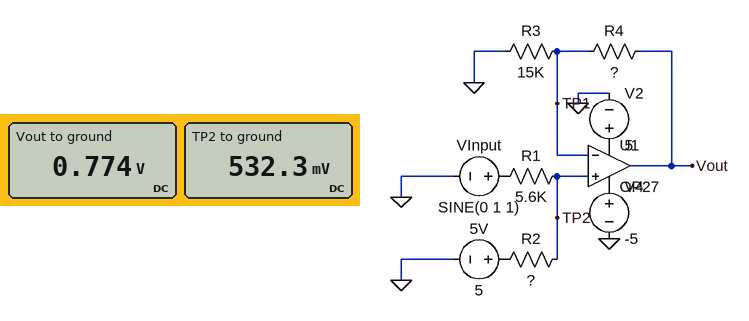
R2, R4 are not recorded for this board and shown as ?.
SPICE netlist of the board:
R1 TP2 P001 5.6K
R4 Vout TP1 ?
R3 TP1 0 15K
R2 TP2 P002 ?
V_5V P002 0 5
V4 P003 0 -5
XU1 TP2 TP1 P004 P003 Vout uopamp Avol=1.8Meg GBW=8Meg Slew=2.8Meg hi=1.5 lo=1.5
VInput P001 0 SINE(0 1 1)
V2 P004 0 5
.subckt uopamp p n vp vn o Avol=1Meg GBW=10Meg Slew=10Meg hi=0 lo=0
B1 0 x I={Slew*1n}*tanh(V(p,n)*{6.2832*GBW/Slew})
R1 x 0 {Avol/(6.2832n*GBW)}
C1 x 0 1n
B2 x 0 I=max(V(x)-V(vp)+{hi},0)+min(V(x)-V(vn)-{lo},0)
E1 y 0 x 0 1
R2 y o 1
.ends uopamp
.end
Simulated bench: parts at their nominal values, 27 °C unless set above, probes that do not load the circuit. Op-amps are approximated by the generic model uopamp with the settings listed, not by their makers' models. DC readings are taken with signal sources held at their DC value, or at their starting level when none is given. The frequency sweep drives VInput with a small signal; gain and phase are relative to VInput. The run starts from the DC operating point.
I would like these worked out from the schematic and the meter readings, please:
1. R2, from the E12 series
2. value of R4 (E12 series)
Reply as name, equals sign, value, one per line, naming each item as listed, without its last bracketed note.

R2, from the E12 series = 47 kΩ
value of R4 = 6.8 kΩ
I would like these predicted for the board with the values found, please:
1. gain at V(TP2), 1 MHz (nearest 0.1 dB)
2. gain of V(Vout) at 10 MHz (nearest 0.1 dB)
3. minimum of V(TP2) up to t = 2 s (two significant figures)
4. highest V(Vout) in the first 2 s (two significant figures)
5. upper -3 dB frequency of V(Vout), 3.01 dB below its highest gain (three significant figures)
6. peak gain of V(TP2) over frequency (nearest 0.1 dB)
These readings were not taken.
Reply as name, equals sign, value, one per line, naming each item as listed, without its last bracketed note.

gain at V(TP2), 1 MHz = -1.0 dB
gain of V(Vout) at 10 MHz = -4.1 dB
minimum of V(TP2) up to t = 2 s = -360 mV
highest V(Vout) in the first 2 s = 2.1 V
upper -3 dB frequency of V(Vout), 3.01 dB below its highest gain = 5.50 MHz
peak gain of V(TP2) over frequency = -1.0 dB
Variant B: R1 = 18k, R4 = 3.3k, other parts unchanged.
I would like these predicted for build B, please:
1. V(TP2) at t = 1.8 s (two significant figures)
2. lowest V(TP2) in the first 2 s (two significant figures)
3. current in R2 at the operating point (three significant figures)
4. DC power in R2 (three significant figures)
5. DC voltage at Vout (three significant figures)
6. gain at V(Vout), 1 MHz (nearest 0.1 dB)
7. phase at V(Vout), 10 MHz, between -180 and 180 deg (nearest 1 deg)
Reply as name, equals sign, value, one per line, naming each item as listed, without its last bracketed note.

V(TP2) at t = 1.8 s = 700 mV
lowest V(TP2) in the first 2 s = 660 mV
current in R2 at the operating point = 76.9 µA
DC power in R2 = 278 µW
DC voltage at Vout = 1.69 V
gain at V(Vout), 1 MHz = -1.2 dB
phase at V(Vout), 10 MHz, between -180 and 180 deg = -57 deg
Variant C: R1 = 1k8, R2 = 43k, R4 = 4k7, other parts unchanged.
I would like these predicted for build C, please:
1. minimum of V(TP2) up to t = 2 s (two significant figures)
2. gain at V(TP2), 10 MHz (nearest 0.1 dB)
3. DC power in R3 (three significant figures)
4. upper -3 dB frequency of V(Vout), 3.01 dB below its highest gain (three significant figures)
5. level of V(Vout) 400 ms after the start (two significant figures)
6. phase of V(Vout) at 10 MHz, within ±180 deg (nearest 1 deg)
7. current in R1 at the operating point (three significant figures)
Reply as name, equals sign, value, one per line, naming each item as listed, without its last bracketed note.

minimum of V(TP2) up to t = 2 s = -760 mV
gain at V(TP2), 10 MHz = -0.4 dB
DC power in R3 = 2.69 µW
upper -3 dB frequency of V(Vout), 3.01 dB below its highest gain = 6.09 MHz
level of V(Vout) 400 ms after the start = 1.0 V
phase of V(Vout) at 10 MHz, within ±180 deg = -59 deg
current in R1 at the operating point = 112 µA
